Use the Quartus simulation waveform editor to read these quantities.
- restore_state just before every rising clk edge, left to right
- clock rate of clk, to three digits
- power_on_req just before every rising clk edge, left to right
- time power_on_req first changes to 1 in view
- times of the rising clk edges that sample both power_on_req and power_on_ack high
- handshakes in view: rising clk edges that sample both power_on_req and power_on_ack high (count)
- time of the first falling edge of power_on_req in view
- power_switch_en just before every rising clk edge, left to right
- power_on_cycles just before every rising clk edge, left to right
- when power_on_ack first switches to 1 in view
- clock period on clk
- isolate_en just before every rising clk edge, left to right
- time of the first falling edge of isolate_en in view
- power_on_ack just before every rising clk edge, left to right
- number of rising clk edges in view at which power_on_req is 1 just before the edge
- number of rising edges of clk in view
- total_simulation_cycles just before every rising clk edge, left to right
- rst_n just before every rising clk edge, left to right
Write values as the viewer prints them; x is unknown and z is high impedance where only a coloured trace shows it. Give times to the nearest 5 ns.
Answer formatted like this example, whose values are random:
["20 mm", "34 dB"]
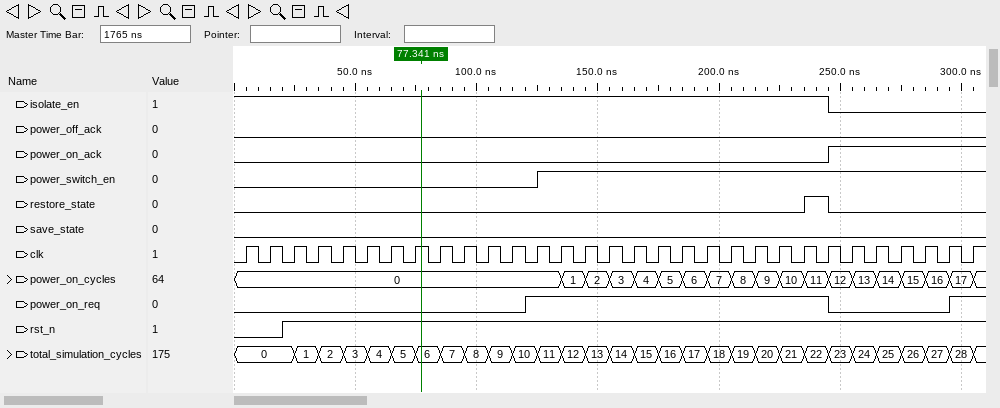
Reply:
["0 0 0 0 0 0 0 0 0 0 0 0 0 0 0 0 0 0 0 0 0 0 0 0 1 0 0 0 0 0 0", "100 MHz", "0 0 0 0 0 0 0 0 0 0 0 0 1 1 1 1 1 1 1 1 1 1 1 1 1 0 0 0 0 0 1", "120 ns", "305 ns", "1", "245 ns", "0 0 0 0 0 0 0 0 0 0 0 0 0 1 1 1 1 1 1 1 1 1 1 1 1 1 1 1 1 1 1", "0, 0, 0, 0, 0, 0, 0, 0, 0, 0, 0, 0, 0, 0, 1, 2, 3, 4, 5, 6, 7, 8, 9, 10, 11, 12, 13, 14, 15, 16, 17", "245 ns", "10 ns", "1 1 1 1 1 1 1 1 1 1 1 1 1 1 1 1 1 1 1 1 1 1 1 1 1 0 0 0 0 0 0", "245 ns", "0 0 0 0 0 0 0 0 0 0 0 0 0 0 0 0 0 0 0 0 0 0 0 0 0 1 1 1 1 1 1", "14", "31", "0, 0, 0, 1, 2, 3, 4, 5, 6, 7, 8, 9, 10, 11, 12, 13, 14, 15, 16, 17, 18, 19, 20, 21, 22, 23, 24, 25, 26, 27, 28", "0 0 1 1 1 1 1 1 1 1 1 1 1 1 1 1 1 1 1 1 1 1 1 1 1 1 1 1 1 1 1"]
